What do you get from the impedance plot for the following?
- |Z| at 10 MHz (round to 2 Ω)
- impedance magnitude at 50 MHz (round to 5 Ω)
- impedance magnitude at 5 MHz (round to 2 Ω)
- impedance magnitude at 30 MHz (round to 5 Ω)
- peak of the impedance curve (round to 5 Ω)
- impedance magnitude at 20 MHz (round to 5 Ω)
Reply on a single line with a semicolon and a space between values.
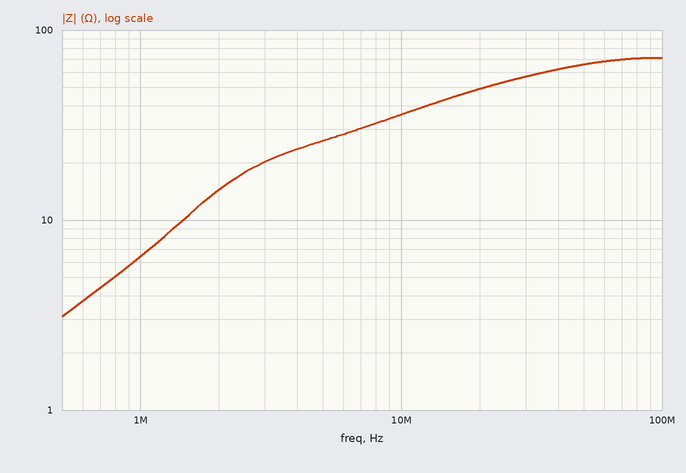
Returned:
36 Ω; 65 Ω; 26 Ω; 55 Ω; 70 Ω; 50 Ω
